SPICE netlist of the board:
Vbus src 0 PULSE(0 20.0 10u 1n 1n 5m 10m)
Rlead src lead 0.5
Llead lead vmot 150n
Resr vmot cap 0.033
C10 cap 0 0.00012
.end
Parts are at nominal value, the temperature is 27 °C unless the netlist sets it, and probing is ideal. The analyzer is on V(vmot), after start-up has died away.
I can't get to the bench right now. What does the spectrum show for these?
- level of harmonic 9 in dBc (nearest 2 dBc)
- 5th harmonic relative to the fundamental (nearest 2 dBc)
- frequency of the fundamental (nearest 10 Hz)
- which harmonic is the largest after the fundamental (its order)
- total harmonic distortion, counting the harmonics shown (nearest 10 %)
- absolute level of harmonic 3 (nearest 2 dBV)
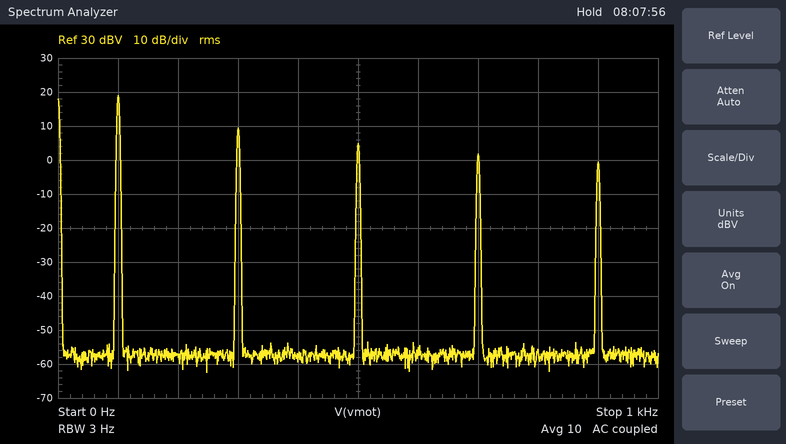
-20 dBc
-14 dBc
100 Hz
3
40 %
10 dBV
